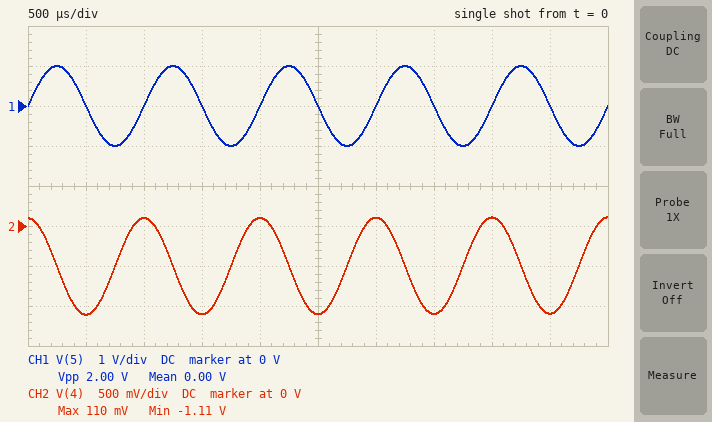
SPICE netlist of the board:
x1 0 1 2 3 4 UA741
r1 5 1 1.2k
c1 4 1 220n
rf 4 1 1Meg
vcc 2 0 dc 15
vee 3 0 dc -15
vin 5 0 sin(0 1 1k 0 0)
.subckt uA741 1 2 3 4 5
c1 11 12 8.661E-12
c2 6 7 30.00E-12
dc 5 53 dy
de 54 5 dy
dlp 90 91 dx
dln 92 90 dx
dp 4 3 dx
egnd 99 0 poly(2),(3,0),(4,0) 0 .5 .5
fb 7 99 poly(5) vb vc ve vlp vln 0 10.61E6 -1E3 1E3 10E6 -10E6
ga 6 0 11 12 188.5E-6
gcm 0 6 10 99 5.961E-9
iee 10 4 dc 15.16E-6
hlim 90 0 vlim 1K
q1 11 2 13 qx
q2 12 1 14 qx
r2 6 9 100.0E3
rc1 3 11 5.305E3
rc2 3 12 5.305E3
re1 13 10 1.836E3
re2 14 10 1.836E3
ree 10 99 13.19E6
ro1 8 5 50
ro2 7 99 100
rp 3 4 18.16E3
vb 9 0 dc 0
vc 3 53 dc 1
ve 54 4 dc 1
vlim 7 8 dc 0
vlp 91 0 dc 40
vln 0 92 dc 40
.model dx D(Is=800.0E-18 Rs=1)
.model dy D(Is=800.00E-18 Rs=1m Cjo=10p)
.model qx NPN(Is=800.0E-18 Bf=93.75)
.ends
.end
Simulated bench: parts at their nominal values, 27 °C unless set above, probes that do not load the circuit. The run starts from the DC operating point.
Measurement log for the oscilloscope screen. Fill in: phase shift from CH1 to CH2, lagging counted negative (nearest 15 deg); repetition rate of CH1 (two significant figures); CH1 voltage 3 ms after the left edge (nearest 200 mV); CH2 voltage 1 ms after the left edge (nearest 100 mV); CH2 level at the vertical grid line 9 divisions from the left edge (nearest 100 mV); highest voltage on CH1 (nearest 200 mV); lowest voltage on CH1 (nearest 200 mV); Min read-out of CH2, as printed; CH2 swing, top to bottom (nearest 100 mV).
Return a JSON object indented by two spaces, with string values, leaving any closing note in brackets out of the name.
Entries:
{
  "phase shift from CH1 to CH2, lagging counted negative": "90 deg",
  "repetition rate of CH1": "1.0 kHz",
  "CH1 voltage 3 ms after the left edge": "0 V",
  "CH2 voltage 1 ms after the left edge": "100 mV",
  "CH2 level at the vertical grid line 9 divisions from the left edge": "-1.1 V",
  "highest voltage on CH1": "1.0 V",
  "lowest voltage on CH1": "-1.0 V",
  "Min read-out of CH2, as printed": "-1.11 V",
  "CH2 swing, top to bottom": "1.2 V"
}
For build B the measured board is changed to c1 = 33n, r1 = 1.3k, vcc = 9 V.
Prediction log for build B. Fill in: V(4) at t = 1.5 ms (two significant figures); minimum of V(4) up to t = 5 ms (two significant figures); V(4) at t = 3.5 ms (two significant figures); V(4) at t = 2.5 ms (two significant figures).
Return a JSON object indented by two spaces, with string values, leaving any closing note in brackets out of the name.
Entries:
{
  "V(4) at t = 1.5 ms": "-7.2 V",
  "minimum of V(4) up to t = 5 ms": "-7.3 V",
  "V(4) at t = 3.5 ms": "-7.0 V",
  "V(4) at t = 2.5 ms": "-7.1 V"
}
